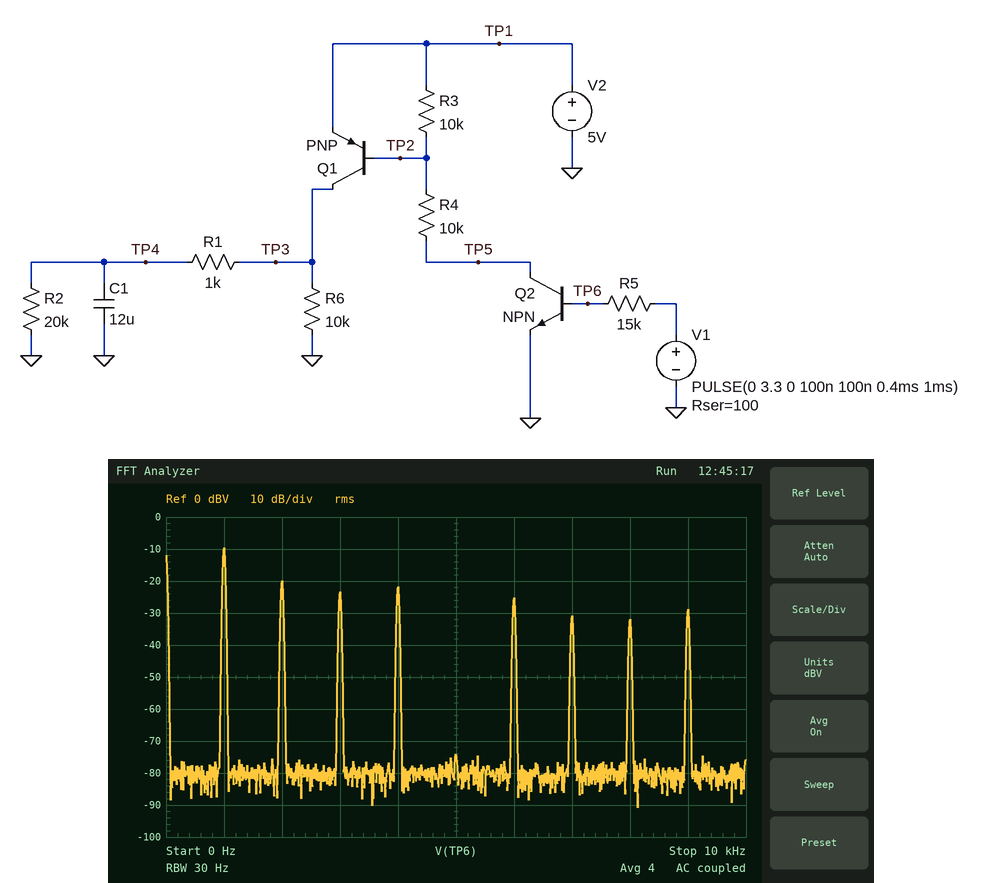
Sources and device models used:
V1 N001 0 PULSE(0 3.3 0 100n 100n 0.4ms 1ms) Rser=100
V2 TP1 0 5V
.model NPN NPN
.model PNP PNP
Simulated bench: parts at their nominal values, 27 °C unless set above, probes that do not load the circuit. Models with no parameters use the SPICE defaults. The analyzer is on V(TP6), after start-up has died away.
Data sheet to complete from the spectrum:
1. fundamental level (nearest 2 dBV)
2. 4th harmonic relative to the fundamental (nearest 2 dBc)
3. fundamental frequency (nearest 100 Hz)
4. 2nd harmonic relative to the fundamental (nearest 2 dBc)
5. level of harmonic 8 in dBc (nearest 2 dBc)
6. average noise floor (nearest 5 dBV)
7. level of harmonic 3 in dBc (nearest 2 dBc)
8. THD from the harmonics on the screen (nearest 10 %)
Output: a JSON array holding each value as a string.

["-10 dBV", "-12 dBc", "1.0 kHz", "-10 dBc", "-22 dBc", "-80 dBV", "-14 dBc", "50 %"]
